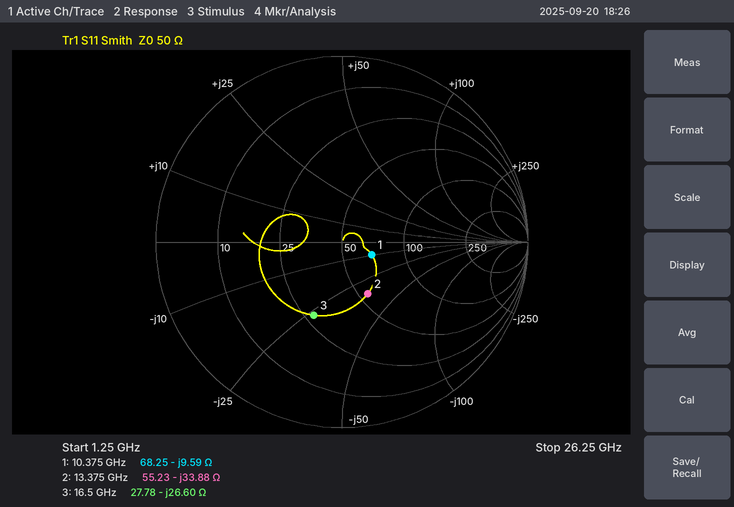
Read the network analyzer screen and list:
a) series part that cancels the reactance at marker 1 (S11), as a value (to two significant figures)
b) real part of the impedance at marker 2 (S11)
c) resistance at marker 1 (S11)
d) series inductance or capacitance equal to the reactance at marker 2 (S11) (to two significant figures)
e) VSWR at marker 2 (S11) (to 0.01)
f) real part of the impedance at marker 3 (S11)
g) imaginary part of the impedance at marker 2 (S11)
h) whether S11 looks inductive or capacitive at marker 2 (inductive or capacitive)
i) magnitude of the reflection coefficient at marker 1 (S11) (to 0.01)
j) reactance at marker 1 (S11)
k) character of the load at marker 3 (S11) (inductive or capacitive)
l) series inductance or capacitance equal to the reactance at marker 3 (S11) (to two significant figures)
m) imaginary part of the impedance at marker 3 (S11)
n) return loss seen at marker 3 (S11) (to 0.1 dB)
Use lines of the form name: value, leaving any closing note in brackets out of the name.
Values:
series part that cancels the reactance at marker 1 (S11), as a value: 150 pH
real part of the impedance at marker 2: 55.23 Ω
resistance at marker 1: 68.25 Ω
series inductance or capacitance equal to the reactance at marker 2 (S11): 350 fF
VSWR at marker 2 (S11): 1.90
real part of the impedance at marker 3: 27.78 Ω
imaginary part of the impedance at marker 2: -33.88 Ω
whether S11 looks inductive or capacitive at marker 2: capacitive
magnitude of the reflection coefficient at marker 1 (S11): 0.17
reactance at marker 1: -9.59 Ω
character of the load at marker 3 (S11): capacitive
series inductance or capacitance equal to the reactance at marker 3 (S11): 360 fF
imaginary part of the impedance at marker 3: -26.60 Ω
return loss seen at marker 3 (S11): 7.5 dB
